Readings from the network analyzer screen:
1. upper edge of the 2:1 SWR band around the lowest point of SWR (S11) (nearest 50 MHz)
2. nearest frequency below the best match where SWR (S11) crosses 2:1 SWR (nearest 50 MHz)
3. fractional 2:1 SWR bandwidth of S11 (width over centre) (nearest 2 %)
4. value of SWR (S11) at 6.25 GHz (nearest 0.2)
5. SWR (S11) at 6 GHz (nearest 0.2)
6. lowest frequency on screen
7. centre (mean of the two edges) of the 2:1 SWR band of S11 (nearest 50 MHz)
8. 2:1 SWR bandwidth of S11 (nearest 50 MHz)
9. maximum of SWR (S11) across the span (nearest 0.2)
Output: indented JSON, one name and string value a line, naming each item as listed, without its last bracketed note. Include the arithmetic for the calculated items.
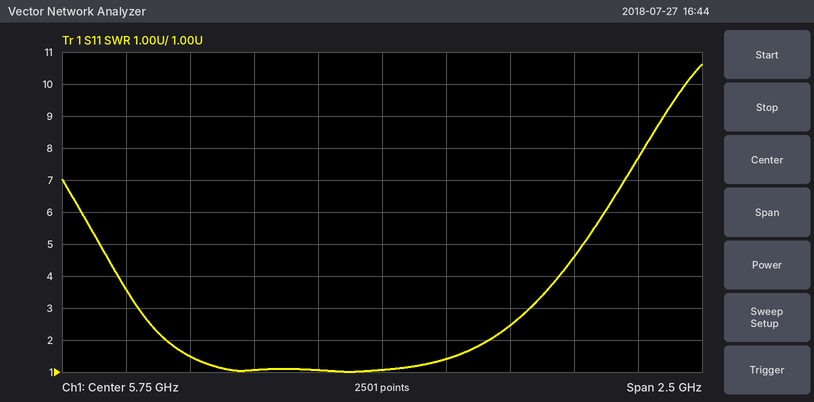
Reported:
{
  "upper edge of the 2:1 SWR band around the lowest point of SWR (S11)": "6.15 GHz",
  "nearest frequency below the best match where SWR (S11) crosses 2:1 SWR": "4.90 GHz",
  "fractional 2:1 SWR bandwidth of S11 (width over centre)": "1.25 GHz / 5.525 GHz ≈ 22.6 %, so 22 % to the nearest 2 %",
  "value of SWR (S11) at 6.25 GHz": "2.4",
  "SWR (S11) at 6 GHz": "1.4",
  "lowest frequency on screen": "4.5 GHz",
  "centre (mean of the two edges) of the 2:1 SWR band of S11": "5.55 GHz",
  "2:1 SWR bandwidth of S11": "6.15 GHz − 4.90 GHz = 1.25 GHz",
  "maximum of SWR (S11) across the span": "10.6"
}
